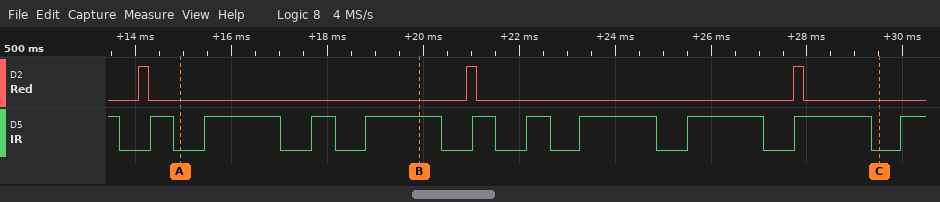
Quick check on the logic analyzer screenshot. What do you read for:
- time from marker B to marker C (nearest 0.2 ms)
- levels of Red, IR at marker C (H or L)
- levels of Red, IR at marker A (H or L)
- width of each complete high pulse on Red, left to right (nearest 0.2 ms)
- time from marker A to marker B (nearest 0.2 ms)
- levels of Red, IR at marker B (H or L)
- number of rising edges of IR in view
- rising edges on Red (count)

9.6 ms
Red=L, IR=L
Red=L, IR=L
0.2 ms, 0.2 ms, 0.2 ms
5 ms
Red=L, IR=H
10
3
